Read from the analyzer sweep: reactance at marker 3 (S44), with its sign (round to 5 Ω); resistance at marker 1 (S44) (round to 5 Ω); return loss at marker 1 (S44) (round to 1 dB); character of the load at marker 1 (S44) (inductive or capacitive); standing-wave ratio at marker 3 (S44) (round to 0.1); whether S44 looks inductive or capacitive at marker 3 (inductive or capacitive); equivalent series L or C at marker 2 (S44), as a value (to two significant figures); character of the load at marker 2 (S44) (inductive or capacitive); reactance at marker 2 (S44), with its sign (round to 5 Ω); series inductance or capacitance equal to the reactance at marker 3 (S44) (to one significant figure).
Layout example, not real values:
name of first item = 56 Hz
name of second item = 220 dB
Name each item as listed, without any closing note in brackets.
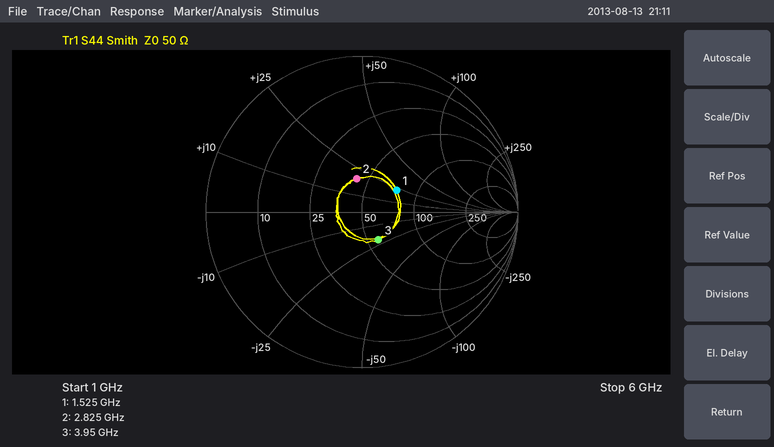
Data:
reactance at marker 3 (S44), with its sign = -20 Ω
resistance at marker 1 (S44) = 75 Ω
return loss at marker 1 (S44) = 12 dB
character of the load at marker 1 (S44) = inductive
standing-wave ratio at marker 3 (S44) = 1.5
whether S44 looks inductive or capacitive at marker 3 = capacitive
equivalent series L or C at marker 2 (S44), as a value = 1.1 nH
character of the load at marker 2 (S44) = inductive
reactance at marker 2 (S44), with its sign = +20 Ω
series inductance or capacitance equal to the reactance at marker 3 (S44) = 2 pF
